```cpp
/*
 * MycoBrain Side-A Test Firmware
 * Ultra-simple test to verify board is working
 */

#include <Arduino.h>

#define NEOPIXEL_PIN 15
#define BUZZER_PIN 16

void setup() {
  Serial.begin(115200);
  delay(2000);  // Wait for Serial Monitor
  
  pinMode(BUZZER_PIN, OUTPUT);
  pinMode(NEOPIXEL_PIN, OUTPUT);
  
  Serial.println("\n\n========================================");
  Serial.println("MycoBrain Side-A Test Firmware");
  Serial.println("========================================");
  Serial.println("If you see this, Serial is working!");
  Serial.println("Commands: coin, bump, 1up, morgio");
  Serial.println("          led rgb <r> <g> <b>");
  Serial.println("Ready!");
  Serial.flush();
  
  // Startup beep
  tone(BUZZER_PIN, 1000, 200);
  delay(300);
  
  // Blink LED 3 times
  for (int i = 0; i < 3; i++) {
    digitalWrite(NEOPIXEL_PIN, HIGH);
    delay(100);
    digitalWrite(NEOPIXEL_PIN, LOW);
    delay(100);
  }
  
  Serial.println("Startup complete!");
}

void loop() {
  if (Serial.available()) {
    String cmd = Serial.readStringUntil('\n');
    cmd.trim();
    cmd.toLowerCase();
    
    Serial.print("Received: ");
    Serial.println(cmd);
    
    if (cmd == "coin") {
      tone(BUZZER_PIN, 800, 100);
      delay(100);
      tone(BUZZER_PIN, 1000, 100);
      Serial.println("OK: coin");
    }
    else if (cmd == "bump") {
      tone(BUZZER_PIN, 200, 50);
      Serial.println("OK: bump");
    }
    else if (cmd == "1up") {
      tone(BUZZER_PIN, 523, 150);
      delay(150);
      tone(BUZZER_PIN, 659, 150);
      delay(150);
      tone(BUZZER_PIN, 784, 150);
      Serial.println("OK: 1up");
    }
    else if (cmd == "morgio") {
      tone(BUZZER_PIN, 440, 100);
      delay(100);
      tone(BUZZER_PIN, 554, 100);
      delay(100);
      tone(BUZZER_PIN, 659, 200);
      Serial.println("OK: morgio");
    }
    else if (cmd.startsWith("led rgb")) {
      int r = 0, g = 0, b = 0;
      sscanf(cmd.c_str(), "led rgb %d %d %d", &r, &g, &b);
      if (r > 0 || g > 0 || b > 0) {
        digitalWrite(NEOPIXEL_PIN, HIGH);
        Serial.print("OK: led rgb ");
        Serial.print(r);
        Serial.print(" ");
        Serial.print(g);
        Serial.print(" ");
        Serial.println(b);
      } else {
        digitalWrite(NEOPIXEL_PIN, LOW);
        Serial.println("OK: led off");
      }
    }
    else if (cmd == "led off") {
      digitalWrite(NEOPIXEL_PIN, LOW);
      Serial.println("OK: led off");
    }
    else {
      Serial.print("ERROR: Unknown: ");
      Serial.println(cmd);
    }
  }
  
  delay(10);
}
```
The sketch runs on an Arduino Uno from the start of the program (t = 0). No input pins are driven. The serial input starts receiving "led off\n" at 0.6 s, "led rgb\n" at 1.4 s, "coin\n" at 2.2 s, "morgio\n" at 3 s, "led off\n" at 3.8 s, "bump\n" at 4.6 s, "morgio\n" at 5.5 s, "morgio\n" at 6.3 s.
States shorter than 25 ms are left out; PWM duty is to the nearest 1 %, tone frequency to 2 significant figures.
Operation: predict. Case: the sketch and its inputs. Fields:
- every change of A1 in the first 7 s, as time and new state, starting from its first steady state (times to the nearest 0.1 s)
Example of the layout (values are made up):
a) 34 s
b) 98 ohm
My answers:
a) 2 s low; 2.3 s high; 2.4 s low; 2.5 s high; 2.6 s low; 2.7 s high; 2.8 s low
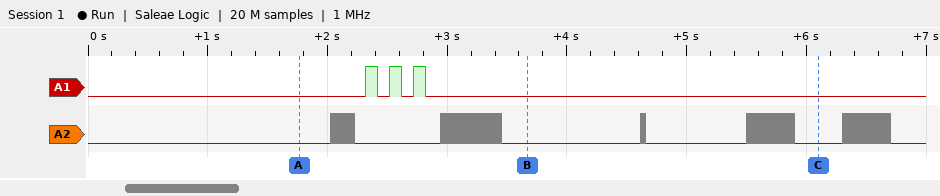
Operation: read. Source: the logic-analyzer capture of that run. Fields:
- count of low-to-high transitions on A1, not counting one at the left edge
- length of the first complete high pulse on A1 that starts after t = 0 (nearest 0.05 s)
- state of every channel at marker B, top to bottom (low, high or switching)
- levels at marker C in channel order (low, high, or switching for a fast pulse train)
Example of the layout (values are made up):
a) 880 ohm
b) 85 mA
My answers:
a) 3
b) 0.10 s
c) A1 low, A2 low
d) A1 low, A2 low
